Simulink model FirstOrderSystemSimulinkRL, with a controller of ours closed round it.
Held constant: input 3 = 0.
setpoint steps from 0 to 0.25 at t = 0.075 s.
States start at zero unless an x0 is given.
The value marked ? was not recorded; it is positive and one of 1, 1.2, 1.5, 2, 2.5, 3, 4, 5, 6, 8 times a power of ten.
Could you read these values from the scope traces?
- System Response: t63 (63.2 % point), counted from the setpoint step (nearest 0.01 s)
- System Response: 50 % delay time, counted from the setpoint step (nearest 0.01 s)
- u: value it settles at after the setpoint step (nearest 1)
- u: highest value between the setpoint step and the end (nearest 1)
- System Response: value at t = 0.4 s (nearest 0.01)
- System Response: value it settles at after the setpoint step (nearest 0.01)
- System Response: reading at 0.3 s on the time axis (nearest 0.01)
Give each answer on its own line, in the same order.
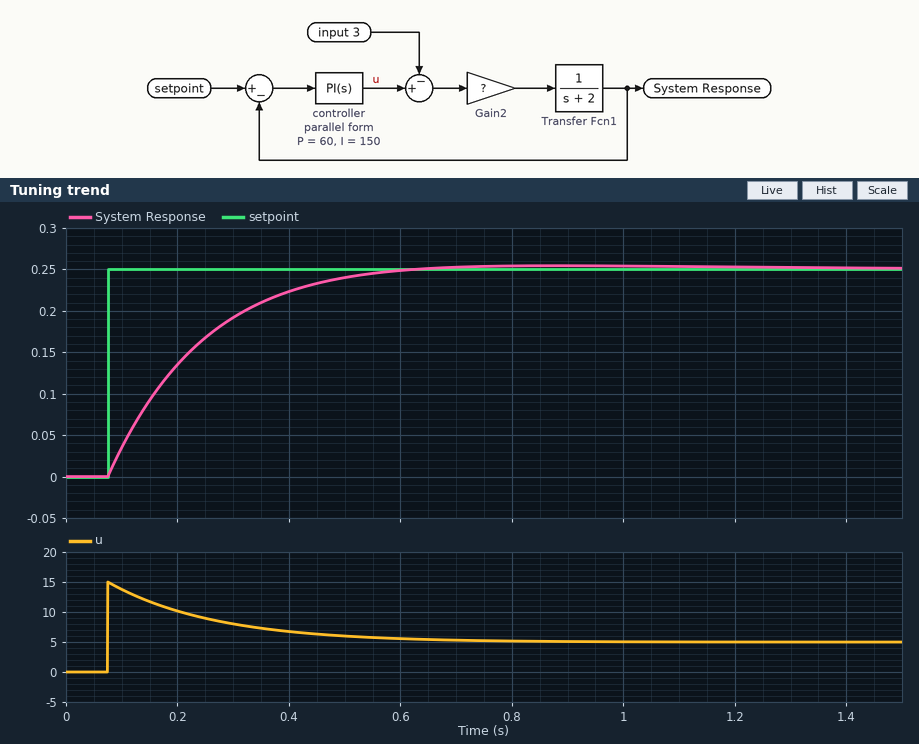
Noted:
0.16 s
0.11 s
5
15
0.22
0.25
0.19
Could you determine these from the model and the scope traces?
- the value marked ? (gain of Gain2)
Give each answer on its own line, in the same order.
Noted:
0.1
